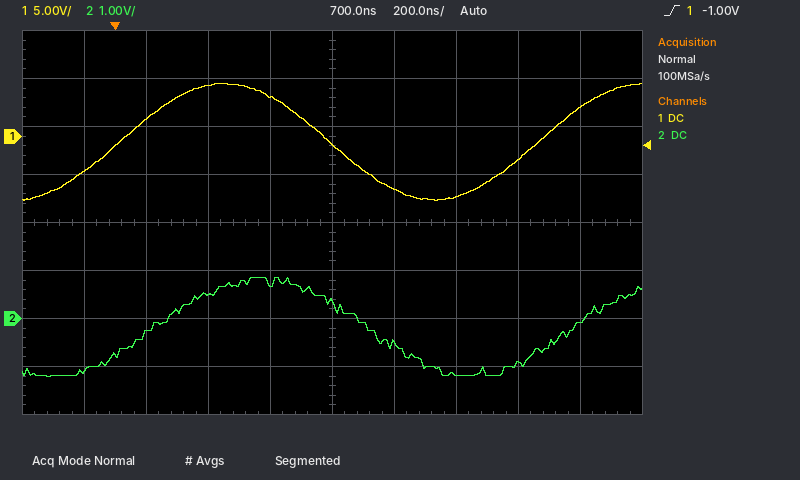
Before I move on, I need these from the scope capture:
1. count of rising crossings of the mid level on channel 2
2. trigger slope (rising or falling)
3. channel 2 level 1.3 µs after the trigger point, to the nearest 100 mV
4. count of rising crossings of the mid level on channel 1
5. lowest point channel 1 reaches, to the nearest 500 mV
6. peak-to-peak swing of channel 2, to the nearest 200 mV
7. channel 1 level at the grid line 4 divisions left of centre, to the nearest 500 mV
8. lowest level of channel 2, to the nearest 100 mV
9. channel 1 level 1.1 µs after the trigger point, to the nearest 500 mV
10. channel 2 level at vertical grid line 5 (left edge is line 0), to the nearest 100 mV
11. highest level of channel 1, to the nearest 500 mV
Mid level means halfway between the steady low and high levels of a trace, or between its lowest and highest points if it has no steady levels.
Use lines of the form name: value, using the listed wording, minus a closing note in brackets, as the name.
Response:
count of rising crossings of the mid level on channel 2: 2
trigger slope: rising
channel 2 level 1.3 µs after the trigger point, to the nearest 100 mV: -900 mV
count of rising crossings of the mid level on channel 1: 2
lowest point channel 1 reaches, to the nearest 500 mV: -6.5 V
peak-to-peak swing of channel 2, to the nearest 200 mV: 2.0 V
channel 1 level at the grid line 4 divisions left of centre, to the nearest 500 mV: -3.5 V
lowest level of channel 2, to the nearest 100 mV: -1.2 V
channel 1 level 1.1 µs after the trigger point, to the nearest 500 mV: -6.5 V
channel 2 level at vertical grid line 5 (left edge is line 0), to the nearest 100 mV: 300 mV
highest level of channel 1, to the nearest 500 mV: 5.5 V
